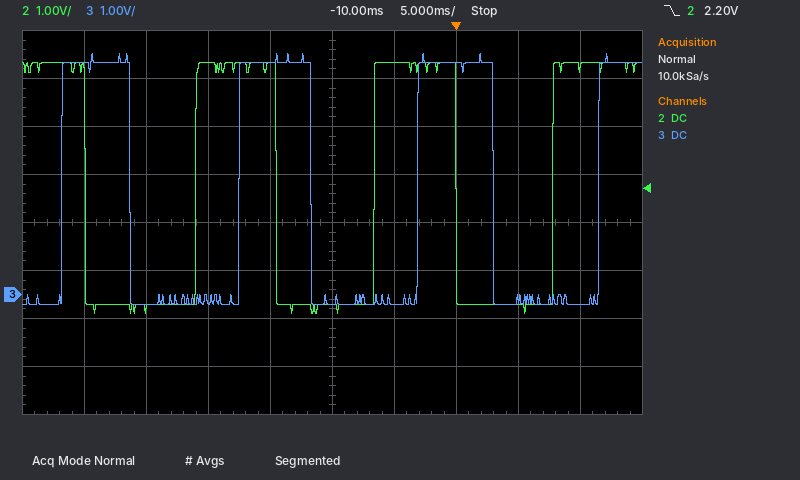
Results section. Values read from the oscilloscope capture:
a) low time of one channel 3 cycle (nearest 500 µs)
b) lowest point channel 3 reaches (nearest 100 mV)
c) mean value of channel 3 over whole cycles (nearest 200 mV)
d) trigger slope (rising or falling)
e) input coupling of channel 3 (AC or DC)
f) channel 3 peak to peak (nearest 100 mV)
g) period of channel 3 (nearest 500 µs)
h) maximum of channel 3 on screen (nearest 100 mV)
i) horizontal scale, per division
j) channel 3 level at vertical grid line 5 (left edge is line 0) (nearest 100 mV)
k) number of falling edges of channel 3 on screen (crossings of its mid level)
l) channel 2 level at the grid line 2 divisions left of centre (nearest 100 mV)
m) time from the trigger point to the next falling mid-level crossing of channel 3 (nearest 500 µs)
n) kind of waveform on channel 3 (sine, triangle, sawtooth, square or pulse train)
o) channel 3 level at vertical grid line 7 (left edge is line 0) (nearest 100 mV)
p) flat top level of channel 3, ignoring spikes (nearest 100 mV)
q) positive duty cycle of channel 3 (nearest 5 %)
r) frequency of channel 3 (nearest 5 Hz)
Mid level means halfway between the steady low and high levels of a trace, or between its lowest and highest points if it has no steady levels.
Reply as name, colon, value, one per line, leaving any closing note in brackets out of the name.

low time of one channel 3 cycle: 8.5 ms
lowest point channel 3 reaches: -200 mV
mean value of channel 3 over whole cycles: 1.8 V
trigger slope: falling
input coupling of channel 3: DC
channel 3 peak to peak: 5.2 V
period of channel 3: 14.5 ms
maximum of channel 3 on screen: 5.0 V
horizontal scale, per division: 5 ms
channel 3 level at vertical grid line 5 (left edge is line 0): -200 mV
number of falling edges of channel 3 on screen: 3
channel 2 level at the grid line 2 divisions left of centre: 4.8 V
time from the trigger point to the next falling mid-level crossing of channel 3: 3.0 ms
kind of waveform on channel 3: pulse train
channel 3 level at vertical grid line 7 (left edge is line 0): 4.8 V
flat top level of channel 3, ignoring spikes: 4.8 V
positive duty cycle of channel 3: 40 %
frequency of channel 3: 70 Hz
